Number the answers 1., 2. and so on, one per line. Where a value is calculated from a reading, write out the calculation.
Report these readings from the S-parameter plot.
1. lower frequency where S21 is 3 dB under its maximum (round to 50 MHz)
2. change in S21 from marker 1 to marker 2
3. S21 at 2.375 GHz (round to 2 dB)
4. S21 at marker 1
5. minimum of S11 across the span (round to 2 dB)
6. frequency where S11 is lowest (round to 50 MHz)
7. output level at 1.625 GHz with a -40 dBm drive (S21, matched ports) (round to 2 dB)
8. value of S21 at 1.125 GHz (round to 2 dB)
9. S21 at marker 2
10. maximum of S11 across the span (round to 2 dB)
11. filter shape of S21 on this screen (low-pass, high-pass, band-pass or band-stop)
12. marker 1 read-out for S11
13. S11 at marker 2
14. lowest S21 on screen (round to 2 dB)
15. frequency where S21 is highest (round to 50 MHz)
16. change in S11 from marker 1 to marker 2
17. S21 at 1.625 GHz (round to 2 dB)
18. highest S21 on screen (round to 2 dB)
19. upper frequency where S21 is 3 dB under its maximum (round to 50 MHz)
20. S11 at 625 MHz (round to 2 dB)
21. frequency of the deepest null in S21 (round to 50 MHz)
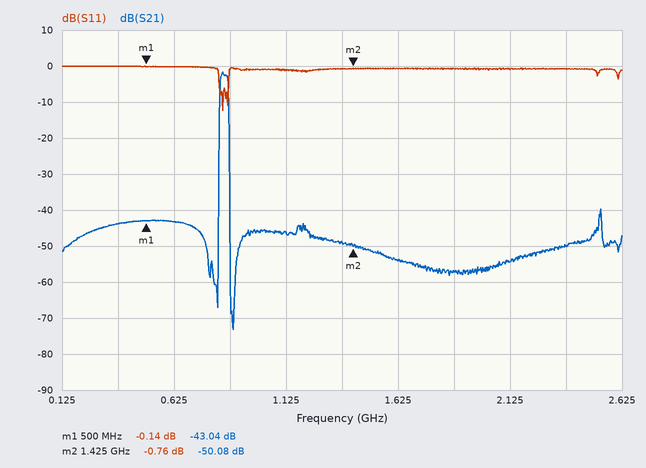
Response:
1. 850 MHz
2. -50.08 − (-43.04) = -7.04 dB
3. -50 dB
4. -43.04 dB
5. -12 dB
6. 850 MHz
7. -40 dBm + (-54 dB) = -94 dBm
8. -46 dB
9. -50.08 dB
10. 0 dB
11. band-pass
12. -0.14 dB
13. -0.76 dB
14. -74 dB
15. 850 MHz
16. -0.76 − (-0.14) = -0.62 dB
17. -54 dB
18. -2 dB
19. 850 MHz
20. 0 dB
21. 900 MHz
